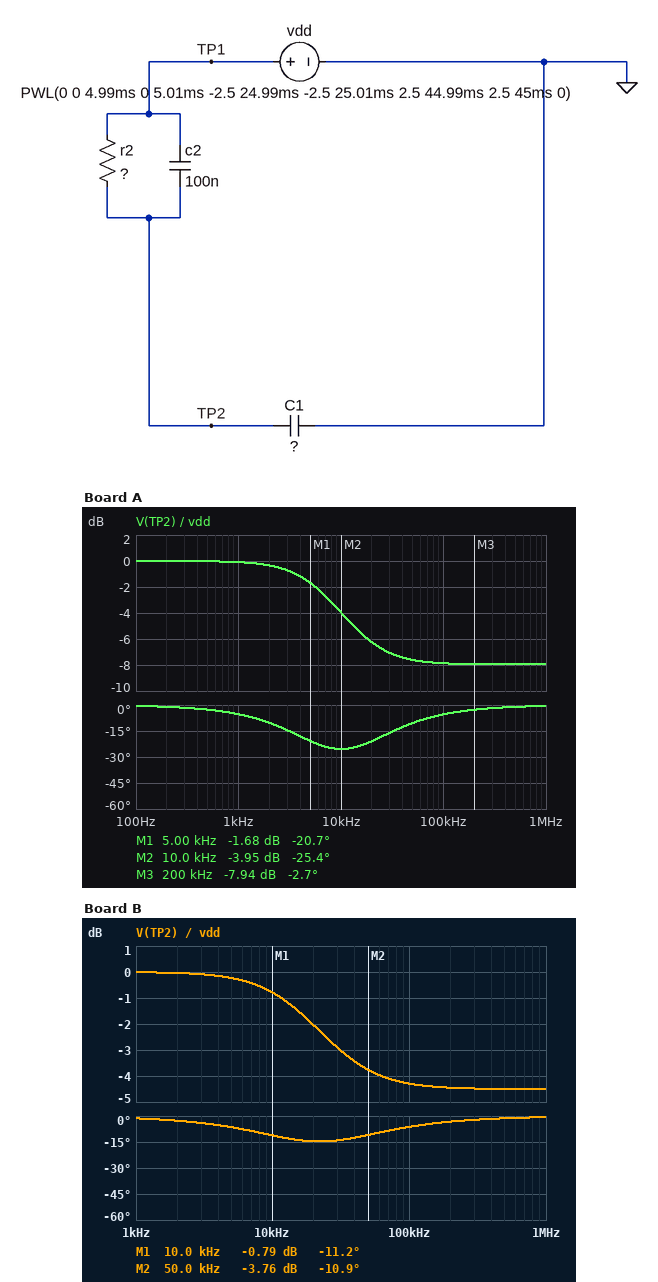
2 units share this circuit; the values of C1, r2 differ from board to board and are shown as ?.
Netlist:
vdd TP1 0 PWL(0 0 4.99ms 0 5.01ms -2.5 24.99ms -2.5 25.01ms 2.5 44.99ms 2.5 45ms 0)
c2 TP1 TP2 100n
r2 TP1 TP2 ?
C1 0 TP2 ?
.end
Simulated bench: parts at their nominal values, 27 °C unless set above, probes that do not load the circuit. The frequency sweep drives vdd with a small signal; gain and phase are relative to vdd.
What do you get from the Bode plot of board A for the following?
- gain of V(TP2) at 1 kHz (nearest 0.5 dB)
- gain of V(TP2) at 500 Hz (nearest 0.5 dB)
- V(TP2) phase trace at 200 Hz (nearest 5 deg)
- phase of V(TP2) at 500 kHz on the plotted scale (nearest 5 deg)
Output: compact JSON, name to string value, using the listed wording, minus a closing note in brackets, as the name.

{"gain of V(TP2) at 1 kHz": "0 dB", "gain of V(TP2) at 500 Hz": "0 dB", "V(TP2) phase trace at 200 Hz": "0 deg", "phase of V(TP2) at 500 kHz on the plotted scale": "0 deg"}
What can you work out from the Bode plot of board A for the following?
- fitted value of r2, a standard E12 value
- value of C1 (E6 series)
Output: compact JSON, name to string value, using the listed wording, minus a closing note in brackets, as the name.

{"fitted value of r2, a standard E12 value": "100 Ω", "value of C1": "150 nF"}
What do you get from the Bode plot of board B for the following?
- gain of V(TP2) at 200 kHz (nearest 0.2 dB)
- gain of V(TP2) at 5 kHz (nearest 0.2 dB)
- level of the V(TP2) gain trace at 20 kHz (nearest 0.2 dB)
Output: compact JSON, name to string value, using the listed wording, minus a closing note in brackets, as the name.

{"gain of V(TP2) at 200 kHz": "-4.4 dB", "gain of V(TP2) at 5 kHz": "-0.2 dB", "level of the V(TP2) gain trace at 20 kHz": "-2.0 dB"}
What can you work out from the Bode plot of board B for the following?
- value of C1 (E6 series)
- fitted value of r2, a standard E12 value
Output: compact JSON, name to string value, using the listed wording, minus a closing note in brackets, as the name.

{"value of C1": "68 nF", "fitted value of r2, a standard E12 value": "56 Ω"}
